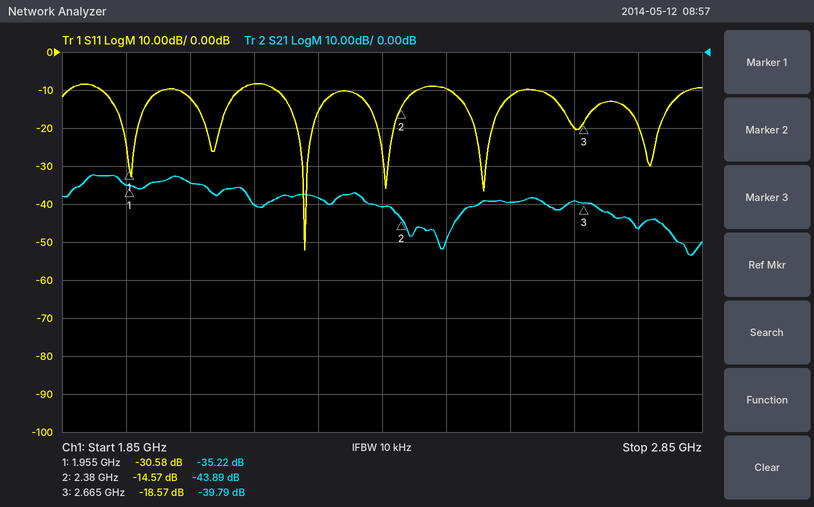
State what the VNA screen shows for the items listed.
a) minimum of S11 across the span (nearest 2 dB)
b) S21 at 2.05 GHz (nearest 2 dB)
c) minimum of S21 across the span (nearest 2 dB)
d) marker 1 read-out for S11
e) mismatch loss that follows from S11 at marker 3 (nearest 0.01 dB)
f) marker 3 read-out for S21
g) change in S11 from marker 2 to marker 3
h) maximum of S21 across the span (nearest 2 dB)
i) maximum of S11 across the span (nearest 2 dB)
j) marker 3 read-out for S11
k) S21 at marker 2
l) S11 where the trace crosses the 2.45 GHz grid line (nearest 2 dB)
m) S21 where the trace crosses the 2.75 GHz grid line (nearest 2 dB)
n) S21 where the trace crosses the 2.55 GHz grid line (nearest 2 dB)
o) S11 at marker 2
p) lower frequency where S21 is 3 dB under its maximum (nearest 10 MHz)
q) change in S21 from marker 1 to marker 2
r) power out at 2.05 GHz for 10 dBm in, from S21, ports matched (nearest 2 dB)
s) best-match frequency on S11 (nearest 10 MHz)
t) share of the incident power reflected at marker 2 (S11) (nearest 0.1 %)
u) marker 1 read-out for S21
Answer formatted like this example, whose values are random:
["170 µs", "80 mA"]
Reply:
["-52 dB", "-34 dB", "-54 dB", "-30.58 dB", "0.06 dB", "-39.79 dB", "-4.00 dB", "-32 dB", "-8 dB", "-18.57 dB", "-43.89 dB", "-10 dB", "-46 dB", "-40 dB", "-14.57 dB", "1.88 GHz", "-8.67 dB", "-24 dBm", "2.23 GHz", "3.5 %", "-35.22 dB"]
